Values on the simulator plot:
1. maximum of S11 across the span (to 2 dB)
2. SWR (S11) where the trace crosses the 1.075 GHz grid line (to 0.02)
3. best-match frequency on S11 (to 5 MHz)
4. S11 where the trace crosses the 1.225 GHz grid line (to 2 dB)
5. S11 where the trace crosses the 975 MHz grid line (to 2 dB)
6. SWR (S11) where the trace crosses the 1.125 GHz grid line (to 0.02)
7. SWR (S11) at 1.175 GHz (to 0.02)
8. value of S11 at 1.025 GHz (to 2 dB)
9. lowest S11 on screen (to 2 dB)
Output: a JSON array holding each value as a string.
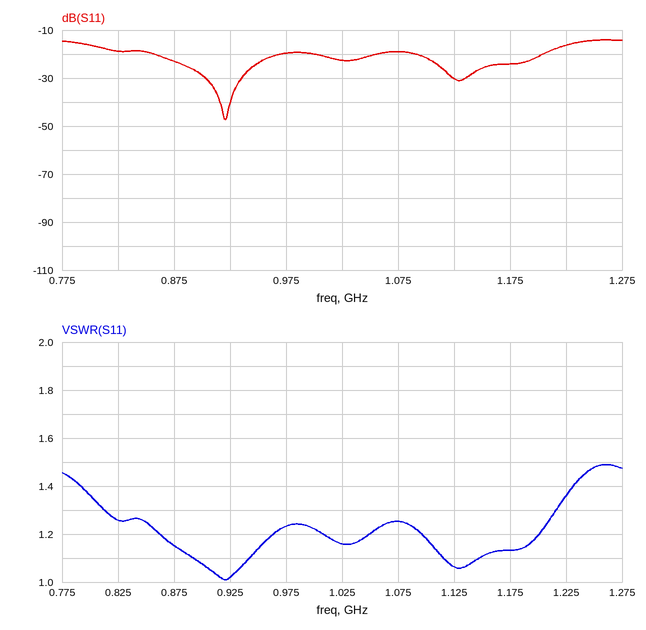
["-14 dB", "1.26", "920 MHz", "-16 dB", "-20 dB", "1.06", "1.14", "-22 dB", "-48 dB"]
